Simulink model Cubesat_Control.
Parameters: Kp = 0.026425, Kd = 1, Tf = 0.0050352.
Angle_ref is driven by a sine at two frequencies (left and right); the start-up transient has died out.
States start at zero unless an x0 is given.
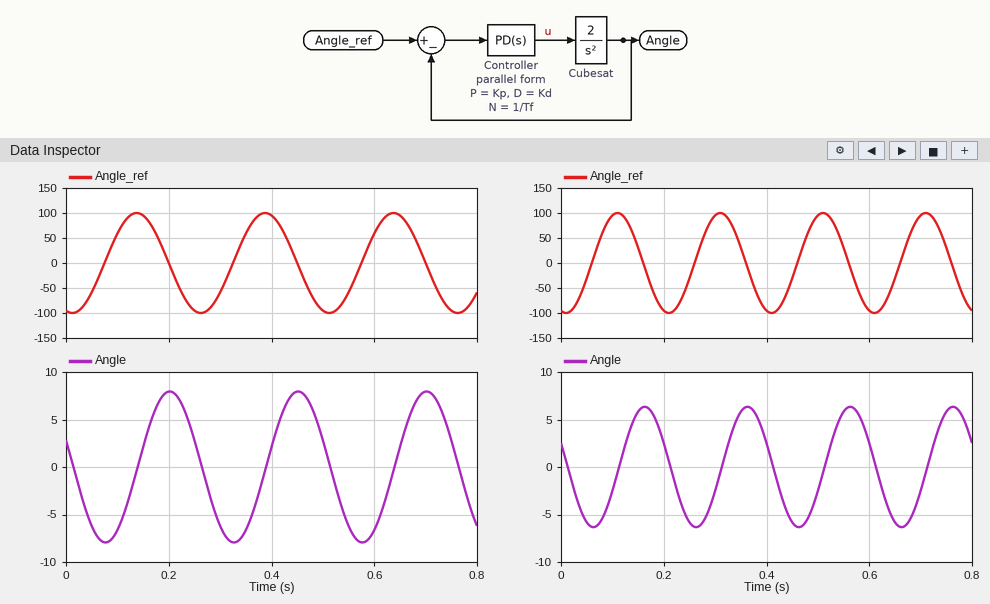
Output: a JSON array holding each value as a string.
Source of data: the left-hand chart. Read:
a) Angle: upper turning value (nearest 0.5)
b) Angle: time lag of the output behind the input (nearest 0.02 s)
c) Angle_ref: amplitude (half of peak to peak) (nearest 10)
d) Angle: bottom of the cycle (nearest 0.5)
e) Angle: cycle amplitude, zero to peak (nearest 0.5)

["8.0", "0.06 s", "100", "-8.0", "8.0"]
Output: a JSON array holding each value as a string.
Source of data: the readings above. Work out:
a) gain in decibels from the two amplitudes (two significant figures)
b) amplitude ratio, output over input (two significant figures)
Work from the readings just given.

["-22 dB", "0.080"]
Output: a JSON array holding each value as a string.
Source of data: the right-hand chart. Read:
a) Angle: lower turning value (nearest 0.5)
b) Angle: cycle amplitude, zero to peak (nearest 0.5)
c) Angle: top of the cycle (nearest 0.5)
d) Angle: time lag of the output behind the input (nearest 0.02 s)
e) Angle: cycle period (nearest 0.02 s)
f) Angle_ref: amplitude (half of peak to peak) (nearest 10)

["-6.5", "6.5", "6.5", "0.06 s", "0.20 s", "100"]
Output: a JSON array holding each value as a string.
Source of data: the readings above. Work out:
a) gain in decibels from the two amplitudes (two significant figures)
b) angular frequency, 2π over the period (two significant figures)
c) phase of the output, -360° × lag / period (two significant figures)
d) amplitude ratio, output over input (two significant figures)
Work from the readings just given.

["-24 dB", "31 rad/s", "-110°", "0.065"]
